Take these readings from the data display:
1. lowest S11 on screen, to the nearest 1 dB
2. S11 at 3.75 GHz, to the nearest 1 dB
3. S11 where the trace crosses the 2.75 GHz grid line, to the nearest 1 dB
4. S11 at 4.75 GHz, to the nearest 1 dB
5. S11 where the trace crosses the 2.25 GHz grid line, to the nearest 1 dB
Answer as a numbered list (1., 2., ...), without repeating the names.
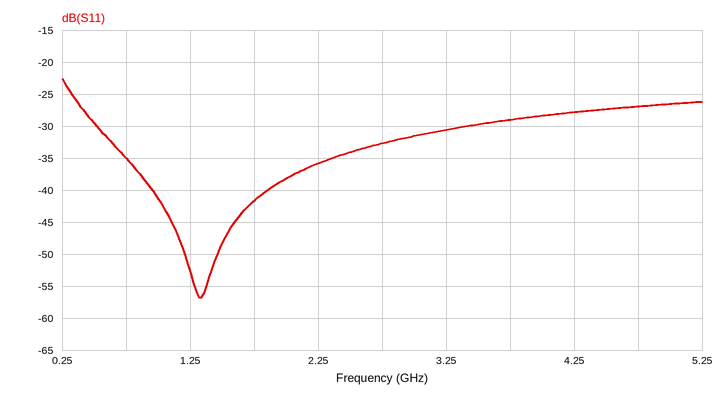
1. -57 dB
2. -29 dB
3. -33 dB
4. -27 dB
5. -36 dB
